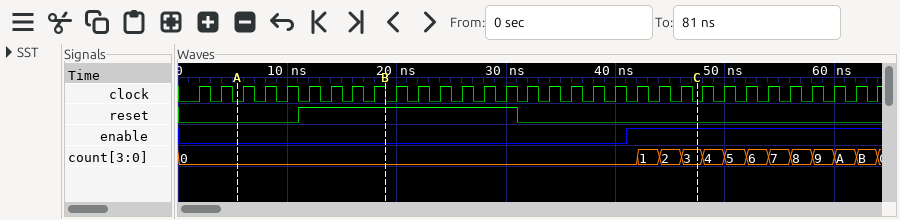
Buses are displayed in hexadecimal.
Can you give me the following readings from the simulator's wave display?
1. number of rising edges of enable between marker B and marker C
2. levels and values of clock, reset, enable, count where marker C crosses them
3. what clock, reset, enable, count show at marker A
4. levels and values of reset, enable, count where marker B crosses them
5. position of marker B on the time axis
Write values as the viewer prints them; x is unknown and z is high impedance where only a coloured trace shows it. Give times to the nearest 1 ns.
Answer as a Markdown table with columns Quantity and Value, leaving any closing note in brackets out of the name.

| Quantity | Value |
|---|---|
| number of rising edges of enable between marker B and marker C | 1 |
| levels and values of clock, reset, enable, count where marker C crosses them | clock=0, reset=0, enable=1, count=3 |
| what clock, reset, enable, count show at marker A | clock=0, reset=0, enable=0, count=0 |
| levels and values of reset, enable, count where marker B crosses them | reset=1, enable=0, count=0 |
| position of marker B on the time axis | 19 ns |
